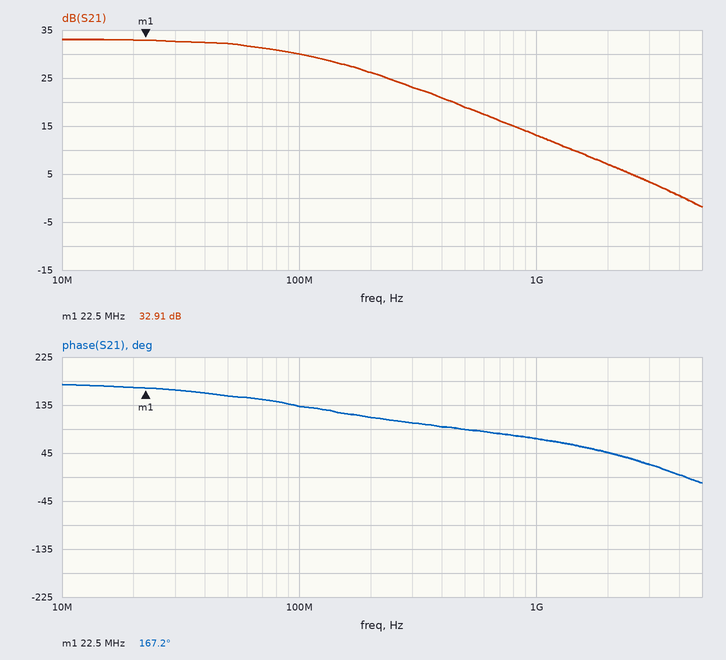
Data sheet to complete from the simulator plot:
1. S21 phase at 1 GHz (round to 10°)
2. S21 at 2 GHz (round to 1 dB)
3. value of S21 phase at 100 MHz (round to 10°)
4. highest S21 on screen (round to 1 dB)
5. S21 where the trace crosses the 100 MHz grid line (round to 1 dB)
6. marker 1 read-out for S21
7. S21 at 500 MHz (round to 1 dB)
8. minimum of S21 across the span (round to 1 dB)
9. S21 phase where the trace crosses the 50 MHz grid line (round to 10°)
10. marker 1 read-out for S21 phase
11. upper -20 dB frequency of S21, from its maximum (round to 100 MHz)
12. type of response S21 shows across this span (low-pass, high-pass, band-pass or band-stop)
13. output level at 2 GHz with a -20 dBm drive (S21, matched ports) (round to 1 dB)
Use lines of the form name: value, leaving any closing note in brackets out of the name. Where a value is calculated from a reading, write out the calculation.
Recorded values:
S21 phase at 1 GHz: 70°
S21 at 2 GHz: 7 dB
value of S21 phase at 100 MHz: 130°
highest S21 on screen: 33 dB
S21 where the trace crosses the 100 MHz grid line: 30 dB
marker 1 read-out for S21: 32.91 dB
S21 at 500 MHz: 19 dB
minimum of S21 across the span: -2 dB
S21 phase where the trace crosses the 50 MHz grid line: 150°
marker 1 read-out for S21 phase: 167.2°
upper -20 dB frequency of S21, from its maximum: 1.0 GHz
type of response S21 shows across this span: low-pass
output level at 2 GHz with a -20 dBm drive (S21, matched ports): -20 dBm + (7 dB) = -13 dBm
